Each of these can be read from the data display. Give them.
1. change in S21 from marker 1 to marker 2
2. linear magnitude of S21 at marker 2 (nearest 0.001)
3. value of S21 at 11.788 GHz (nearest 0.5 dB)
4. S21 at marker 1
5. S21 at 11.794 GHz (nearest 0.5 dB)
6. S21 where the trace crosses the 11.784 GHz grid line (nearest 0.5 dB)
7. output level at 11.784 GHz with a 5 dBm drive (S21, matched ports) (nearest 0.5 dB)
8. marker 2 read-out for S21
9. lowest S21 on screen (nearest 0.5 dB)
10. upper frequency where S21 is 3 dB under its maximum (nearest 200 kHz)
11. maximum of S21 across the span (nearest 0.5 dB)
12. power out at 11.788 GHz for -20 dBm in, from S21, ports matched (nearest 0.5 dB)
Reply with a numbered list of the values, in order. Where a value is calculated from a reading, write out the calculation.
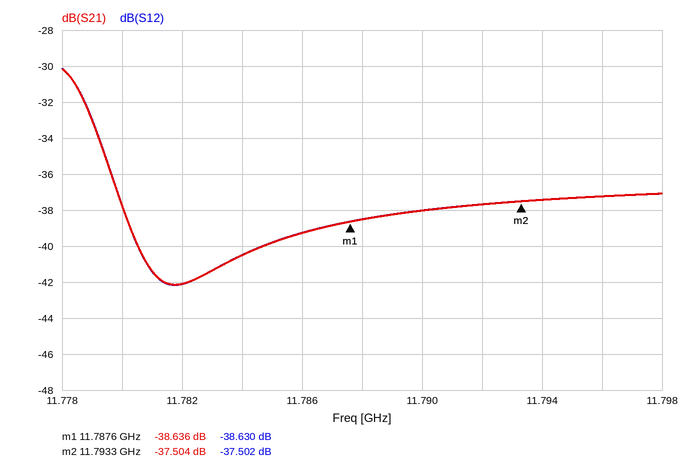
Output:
1. -37.504 − (-38.636) = 1.132 dB
2. 10^(-37.504/20) ≈ 0.013
3. -38.5 dB
4. -38.636 dB
5. -37.5 dB
6. -40.5 dB
7. 5 dBm + (-40.5 dB) = -35.5 dBm
8. -37.504 dB
9. -42.0 dB
10. 11.7790 GHz
11. -30.0 dB
12. -20 dBm + (-38.5 dB) = -58.5 dBm
